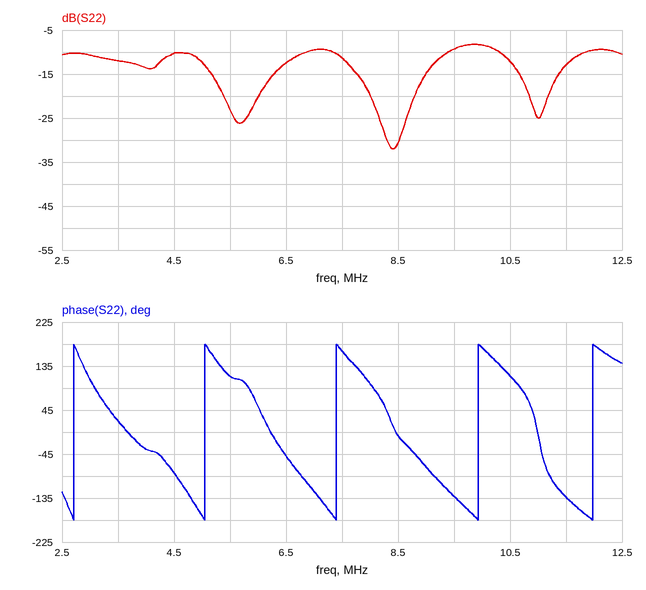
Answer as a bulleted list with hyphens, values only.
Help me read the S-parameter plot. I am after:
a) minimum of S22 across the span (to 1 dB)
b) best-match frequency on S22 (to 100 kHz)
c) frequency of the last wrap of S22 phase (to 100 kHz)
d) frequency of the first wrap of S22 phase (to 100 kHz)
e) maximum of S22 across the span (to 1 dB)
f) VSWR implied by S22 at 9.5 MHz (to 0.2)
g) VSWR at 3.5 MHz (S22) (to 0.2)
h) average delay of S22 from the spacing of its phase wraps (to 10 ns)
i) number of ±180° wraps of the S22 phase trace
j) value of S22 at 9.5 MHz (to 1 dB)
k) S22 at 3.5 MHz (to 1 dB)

- -32 dB
- 8.4 MHz
- 12.0 MHz
- 2.7 MHz
- -8 dB
- 2.0
- 1.6
- 430 ns
- 5
- -9 dB
- -12 dB
